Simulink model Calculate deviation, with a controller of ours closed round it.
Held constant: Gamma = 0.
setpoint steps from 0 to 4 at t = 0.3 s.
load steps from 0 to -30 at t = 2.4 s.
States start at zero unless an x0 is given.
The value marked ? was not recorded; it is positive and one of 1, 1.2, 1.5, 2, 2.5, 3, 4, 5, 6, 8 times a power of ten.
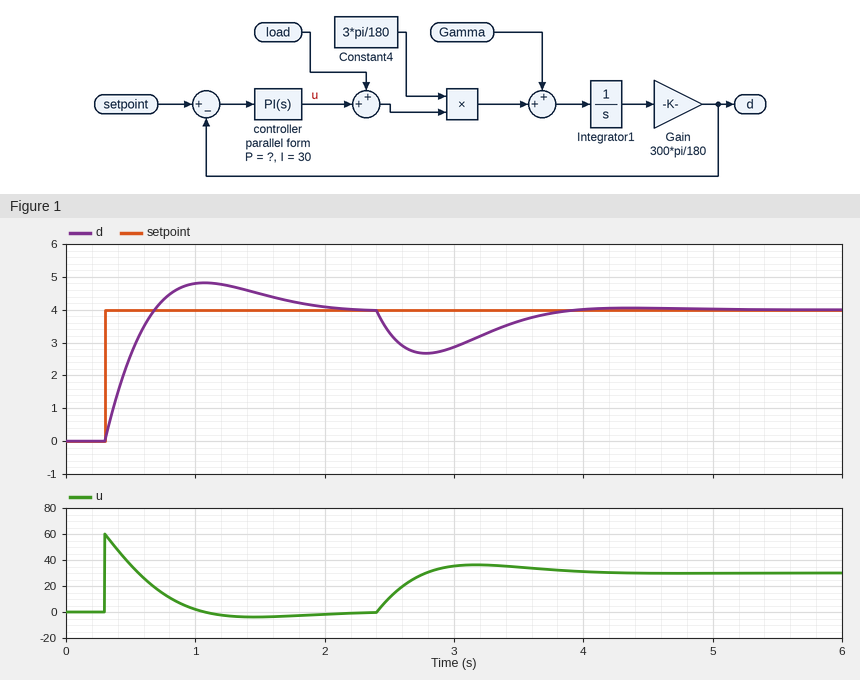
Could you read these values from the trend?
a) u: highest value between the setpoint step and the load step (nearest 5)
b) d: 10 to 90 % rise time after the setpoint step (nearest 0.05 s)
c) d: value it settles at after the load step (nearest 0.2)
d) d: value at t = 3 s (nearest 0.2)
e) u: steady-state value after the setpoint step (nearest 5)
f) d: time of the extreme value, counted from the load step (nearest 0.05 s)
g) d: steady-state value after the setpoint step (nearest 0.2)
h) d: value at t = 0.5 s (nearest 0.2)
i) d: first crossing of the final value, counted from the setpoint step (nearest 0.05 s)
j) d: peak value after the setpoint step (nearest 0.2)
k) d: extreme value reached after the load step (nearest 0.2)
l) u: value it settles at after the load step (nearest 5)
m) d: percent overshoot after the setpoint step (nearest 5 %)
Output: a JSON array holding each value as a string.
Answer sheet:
["60", "0.30 s", "4.0", "2.8", "0", "0.40 s", "4.0", "2.6", "0.40 s", "4.8", "2.6", "30", "20 %"]
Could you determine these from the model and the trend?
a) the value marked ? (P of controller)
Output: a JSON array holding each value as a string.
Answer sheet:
["15"]
